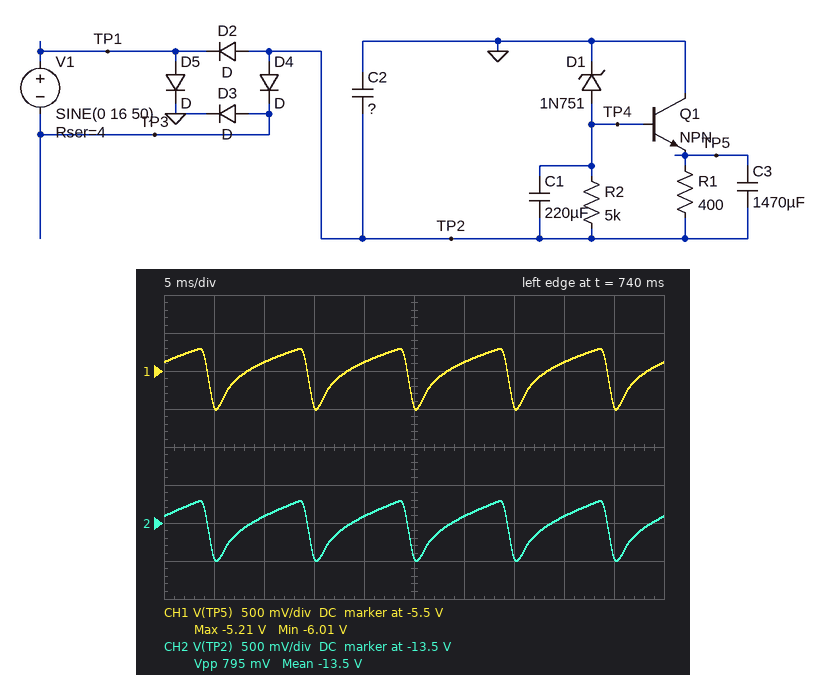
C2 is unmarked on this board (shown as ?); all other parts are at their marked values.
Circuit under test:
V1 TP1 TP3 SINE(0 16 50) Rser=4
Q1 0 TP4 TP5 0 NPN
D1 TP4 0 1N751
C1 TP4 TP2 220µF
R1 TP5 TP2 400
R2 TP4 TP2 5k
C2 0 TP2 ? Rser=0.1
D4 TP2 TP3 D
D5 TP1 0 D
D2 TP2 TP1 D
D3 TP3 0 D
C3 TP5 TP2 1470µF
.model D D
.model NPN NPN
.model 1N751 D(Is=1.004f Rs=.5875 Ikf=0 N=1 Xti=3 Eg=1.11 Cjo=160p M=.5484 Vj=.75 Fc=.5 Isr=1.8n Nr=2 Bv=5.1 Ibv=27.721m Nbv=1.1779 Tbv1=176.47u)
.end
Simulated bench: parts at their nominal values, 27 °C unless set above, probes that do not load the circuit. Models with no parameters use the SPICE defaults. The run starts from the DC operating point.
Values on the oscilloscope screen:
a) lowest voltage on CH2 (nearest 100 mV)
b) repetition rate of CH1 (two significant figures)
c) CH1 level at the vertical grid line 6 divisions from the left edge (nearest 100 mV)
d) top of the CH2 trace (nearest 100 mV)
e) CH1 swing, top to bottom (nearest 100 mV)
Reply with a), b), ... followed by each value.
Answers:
a) -14.0 V
b) 100 Hz
c) -5.4 V
d) -13.2 V
e) 800 mV
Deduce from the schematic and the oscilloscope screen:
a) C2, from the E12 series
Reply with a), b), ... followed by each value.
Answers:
a) 180 µF
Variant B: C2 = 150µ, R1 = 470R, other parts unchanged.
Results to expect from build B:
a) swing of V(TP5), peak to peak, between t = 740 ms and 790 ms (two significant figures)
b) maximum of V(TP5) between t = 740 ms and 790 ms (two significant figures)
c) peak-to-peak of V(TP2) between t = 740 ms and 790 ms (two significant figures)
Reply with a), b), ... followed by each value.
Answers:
a) 850 mV
b) -5.2 V
c) 840 mV
